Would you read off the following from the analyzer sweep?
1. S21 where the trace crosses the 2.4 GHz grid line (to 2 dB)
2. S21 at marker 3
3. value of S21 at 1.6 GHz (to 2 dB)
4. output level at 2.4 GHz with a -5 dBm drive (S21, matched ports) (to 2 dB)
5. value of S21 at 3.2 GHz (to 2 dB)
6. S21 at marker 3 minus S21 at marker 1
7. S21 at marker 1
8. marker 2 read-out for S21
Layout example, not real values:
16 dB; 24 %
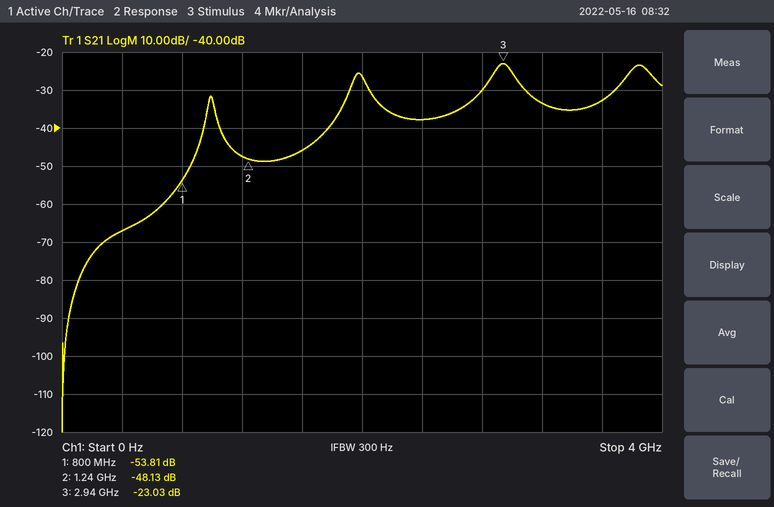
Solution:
-38 dB; -23.03 dB; -46 dB; -42 dBm; -34 dB; 30.78 dB; -53.81 dB; -48.13 dB
